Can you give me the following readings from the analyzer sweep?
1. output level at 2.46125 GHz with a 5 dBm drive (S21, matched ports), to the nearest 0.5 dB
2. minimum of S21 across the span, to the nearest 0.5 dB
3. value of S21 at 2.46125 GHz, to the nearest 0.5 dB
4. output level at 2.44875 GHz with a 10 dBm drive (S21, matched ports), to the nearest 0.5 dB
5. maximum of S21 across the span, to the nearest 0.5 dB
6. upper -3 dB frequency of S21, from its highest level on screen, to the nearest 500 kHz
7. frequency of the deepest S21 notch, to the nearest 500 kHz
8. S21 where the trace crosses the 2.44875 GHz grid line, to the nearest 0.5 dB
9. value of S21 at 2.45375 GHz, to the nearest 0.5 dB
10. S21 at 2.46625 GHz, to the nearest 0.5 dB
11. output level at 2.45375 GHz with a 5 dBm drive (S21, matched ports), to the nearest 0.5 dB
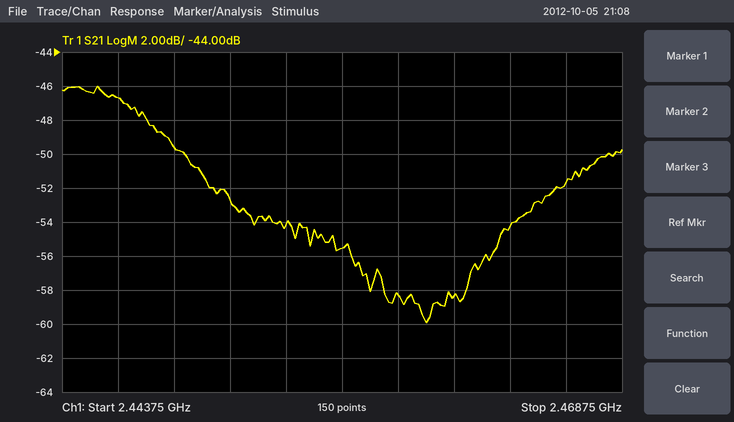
-53.5 dBm
-60.0 dB
-58.5 dB
-39.5 dBm
-46.0 dB
2.4485 GHz
2.4600 GHz
-49.5 dB
-54.0 dB
-51.5 dB
-49.0 dBm
